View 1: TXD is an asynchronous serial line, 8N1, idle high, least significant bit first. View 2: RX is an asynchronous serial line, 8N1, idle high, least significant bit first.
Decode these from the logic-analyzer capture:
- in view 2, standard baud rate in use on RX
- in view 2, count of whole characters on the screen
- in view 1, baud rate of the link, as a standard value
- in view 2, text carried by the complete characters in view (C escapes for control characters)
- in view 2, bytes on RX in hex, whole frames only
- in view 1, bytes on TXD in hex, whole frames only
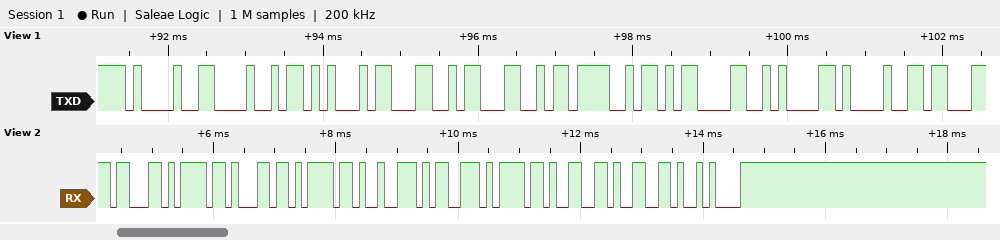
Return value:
9600 baud
10
9600 baud
"colorsoff\n"
0x63 0x6F 0x6C 0x6F 0x72 0x73 0x6F 0x66 0x66 0x0A
21 48 45 4C 4C 4F 0D 0A 21
